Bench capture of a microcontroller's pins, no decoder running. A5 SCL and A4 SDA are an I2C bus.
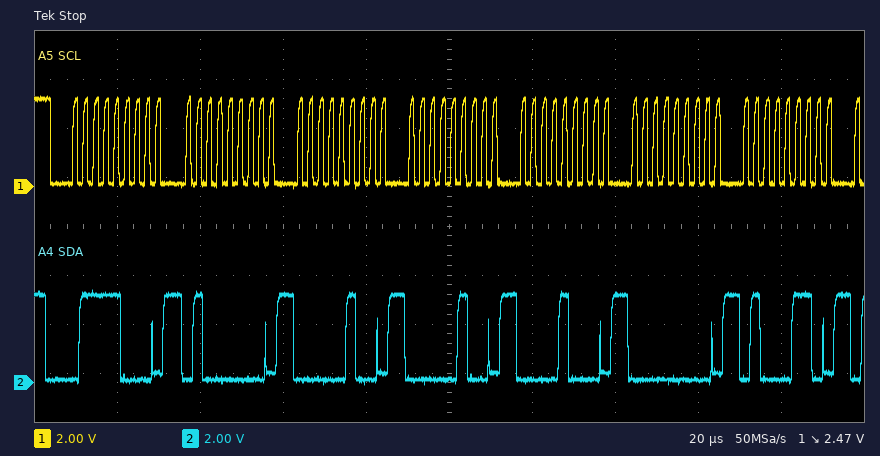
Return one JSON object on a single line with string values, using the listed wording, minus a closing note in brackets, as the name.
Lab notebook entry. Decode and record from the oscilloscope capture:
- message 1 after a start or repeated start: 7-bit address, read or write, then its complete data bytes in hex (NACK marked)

{"message 1 after a start or repeated start: 7-bit address, read or write, then its complete data bytes in hex": "0x3C write: 40 04 04 08 00 46"}
